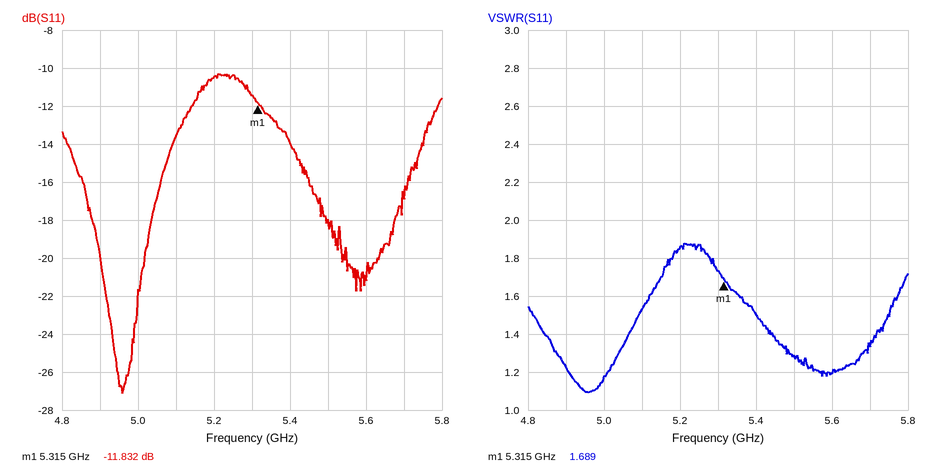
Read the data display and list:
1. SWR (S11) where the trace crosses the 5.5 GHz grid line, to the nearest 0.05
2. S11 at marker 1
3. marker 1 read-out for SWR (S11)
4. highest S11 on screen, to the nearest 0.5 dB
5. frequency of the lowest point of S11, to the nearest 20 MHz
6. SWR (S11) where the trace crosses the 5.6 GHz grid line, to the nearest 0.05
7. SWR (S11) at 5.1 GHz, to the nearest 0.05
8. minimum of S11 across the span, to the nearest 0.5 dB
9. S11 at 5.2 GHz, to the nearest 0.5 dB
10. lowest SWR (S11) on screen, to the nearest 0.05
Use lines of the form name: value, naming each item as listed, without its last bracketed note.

SWR (S11) where the trace crosses the 5.5 GHz grid line, to the nearest 0.05: 1.30
S11 at marker 1: -11.832 dB
marker 1 read-out for SWR: 1.689
highest S11 on screen, to the nearest 0.5 dB: -10.5 dB
frequency of the lowest point of S11, to the nearest 20 MHz: 4.96 GHz
SWR (S11) where the trace crosses the 5.6 GHz grid line, to the nearest 0.05: 1.20
SWR (S11) at 5.1 GHz, to the nearest 0.05: 1.55
minimum of S11 across the span, to the nearest 0.5 dB: -27.0 dB
S11 at 5.2 GHz, to the nearest 0.5 dB: -10.5 dB
lowest SWR (S11) on screen, to the nearest 0.05: 1.10
